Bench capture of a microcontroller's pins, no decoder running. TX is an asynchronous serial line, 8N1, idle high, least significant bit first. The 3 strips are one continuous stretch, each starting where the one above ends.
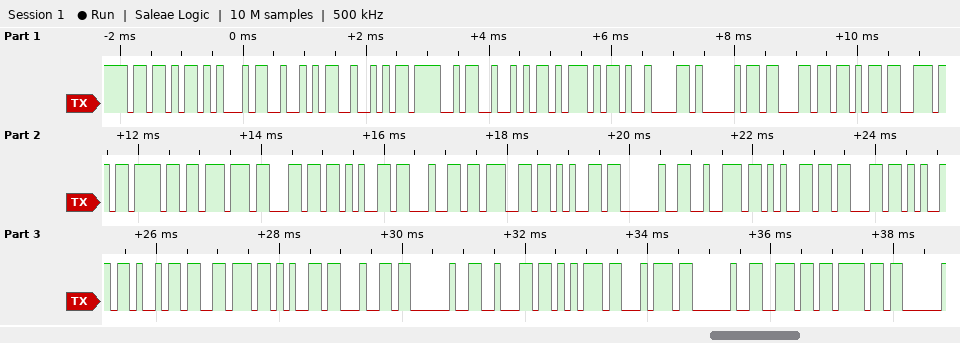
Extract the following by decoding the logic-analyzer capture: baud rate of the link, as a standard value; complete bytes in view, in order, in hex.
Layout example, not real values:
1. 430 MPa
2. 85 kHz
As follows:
1. 9600 baud
2. 5B 45 52 52 4F 52 5D 09 41 63 6B 6E 6F 77 6C 65 64 67 65 20 72 65 63 65 69 76 65 64 20 62 75 74 20 6E 6F
